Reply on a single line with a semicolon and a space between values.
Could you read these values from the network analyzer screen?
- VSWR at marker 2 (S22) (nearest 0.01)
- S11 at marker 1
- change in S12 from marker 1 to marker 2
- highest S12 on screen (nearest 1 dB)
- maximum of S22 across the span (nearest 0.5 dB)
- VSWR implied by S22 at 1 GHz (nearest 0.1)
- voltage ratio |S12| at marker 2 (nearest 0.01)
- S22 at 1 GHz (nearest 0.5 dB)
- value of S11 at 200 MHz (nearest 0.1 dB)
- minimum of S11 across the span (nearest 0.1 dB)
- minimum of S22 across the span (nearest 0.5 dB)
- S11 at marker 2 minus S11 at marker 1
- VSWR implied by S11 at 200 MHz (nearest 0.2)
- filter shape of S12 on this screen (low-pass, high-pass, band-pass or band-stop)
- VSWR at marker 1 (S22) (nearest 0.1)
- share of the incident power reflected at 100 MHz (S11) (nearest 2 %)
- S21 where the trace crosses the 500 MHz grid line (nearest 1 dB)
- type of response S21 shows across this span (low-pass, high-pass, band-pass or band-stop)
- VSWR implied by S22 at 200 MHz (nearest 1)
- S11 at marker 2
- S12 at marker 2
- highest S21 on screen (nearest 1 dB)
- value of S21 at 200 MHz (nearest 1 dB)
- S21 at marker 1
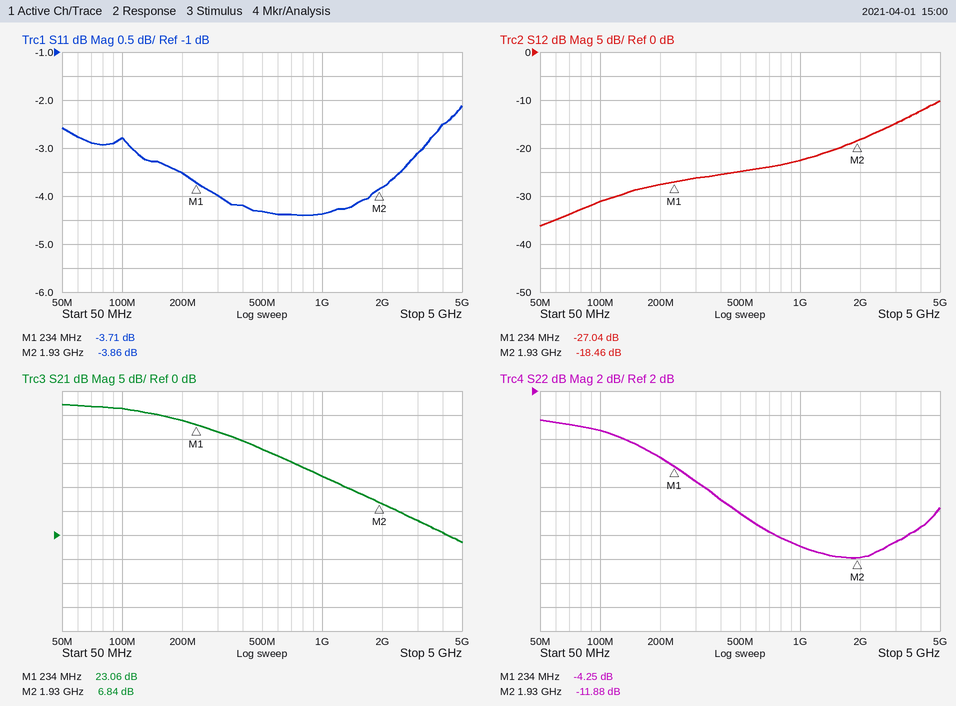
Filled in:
1.68; -3.71 dB; 8.58 dB; -10 dB; -0.5 dB; 1.8; 0.12; -11.0 dB; -3.5 dB; -4.4 dB; -12.0 dB; -0.15 dB; 5.0; high-pass; 4.2; 52 %; 18 dB; low-pass; 5; -3.86 dB; -18.46 dB; 27 dB; 24 dB; 23.06 dB
